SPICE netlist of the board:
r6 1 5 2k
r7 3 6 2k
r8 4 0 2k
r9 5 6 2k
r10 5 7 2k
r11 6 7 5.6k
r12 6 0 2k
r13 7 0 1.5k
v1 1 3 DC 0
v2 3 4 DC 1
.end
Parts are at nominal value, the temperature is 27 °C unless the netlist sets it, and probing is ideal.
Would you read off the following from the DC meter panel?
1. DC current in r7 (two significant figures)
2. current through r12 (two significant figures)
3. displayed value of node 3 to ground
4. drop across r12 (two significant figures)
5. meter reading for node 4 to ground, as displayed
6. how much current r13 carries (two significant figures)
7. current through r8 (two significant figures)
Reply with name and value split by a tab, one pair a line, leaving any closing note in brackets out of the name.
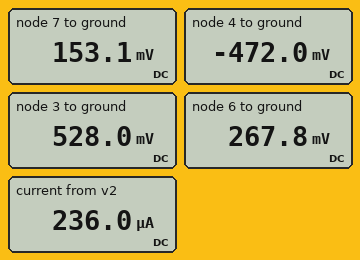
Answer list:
DC current in r7	130 µA
current through r12	130 µA
displayed value of node 3 to ground	528.0 mV
drop across r12	270 mV
meter reading for node 4 to ground, as displayed	-472.0 mV
how much current r13 carries	100 µA
current through r8	240 µA
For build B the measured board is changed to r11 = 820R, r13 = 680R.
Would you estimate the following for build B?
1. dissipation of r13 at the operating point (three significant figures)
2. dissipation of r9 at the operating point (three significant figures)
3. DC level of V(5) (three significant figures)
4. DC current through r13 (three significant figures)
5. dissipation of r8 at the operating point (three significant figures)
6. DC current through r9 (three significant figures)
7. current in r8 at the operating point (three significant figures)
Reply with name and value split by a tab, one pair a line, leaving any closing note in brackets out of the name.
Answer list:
dissipation of r13 at the operating point	18.6 µW
dissipation of r9 at the operating point	2.71 µW
DC level of V(5)	261 mV
DC current through r13	165 µA
dissipation of r8 at the operating point	134 µW
DC current through r9	36.8 µA
current in r8 at the operating point	259 µA
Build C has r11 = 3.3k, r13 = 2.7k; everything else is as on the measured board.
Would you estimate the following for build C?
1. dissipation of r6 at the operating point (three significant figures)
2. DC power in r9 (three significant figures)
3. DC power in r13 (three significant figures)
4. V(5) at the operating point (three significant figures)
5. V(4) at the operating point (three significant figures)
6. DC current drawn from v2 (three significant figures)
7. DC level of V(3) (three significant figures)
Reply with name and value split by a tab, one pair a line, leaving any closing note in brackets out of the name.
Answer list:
dissipation of r6 at the operating point	18.8 µW
DC power in r9	2.15 µW
DC power in r13	18.7 µW
V(5) at the operating point	353 mV
V(4) at the operating point	-453 mV
DC current drawn from v2	227 µA
DC level of V(3)	547 mV
